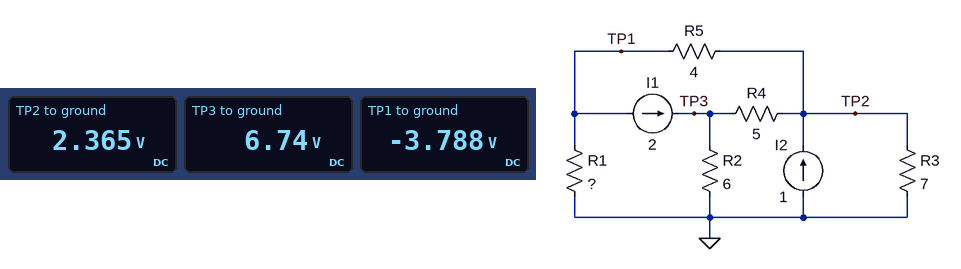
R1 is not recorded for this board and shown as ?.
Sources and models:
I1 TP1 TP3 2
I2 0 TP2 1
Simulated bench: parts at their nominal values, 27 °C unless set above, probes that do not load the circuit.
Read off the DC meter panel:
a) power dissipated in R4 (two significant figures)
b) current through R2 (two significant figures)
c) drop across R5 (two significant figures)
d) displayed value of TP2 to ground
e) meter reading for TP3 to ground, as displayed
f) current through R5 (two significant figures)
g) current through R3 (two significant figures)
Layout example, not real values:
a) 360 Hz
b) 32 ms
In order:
a) 3.8 W
b) 1.1 A
c) 6.2 V
d) 2.365 V
e) 6.74 V
f) 1.5 A
g) 340 mA
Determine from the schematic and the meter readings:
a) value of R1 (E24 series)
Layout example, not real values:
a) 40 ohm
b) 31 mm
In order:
a) 8.2 Ω
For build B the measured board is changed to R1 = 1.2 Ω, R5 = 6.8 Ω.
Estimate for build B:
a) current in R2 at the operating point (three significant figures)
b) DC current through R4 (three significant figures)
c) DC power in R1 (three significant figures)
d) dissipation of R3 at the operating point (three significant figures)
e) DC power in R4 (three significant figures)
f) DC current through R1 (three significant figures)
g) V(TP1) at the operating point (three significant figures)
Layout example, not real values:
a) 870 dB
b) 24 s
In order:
a) 1.36 A
b) 637 mA
c) 1.39 W
d) 3.56 W
e) 2.03 W
f) 1.08 A
g) -1.29 V
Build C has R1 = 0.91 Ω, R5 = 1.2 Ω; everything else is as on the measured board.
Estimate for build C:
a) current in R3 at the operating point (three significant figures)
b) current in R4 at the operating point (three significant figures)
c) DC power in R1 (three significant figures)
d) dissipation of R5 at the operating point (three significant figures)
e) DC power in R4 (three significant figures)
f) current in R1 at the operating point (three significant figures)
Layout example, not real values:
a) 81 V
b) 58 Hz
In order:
a) 248 mA
b) 933 mA
c) 90.2 mW
d) 3.41 W
e) 4.35 W
f) 315 mA
